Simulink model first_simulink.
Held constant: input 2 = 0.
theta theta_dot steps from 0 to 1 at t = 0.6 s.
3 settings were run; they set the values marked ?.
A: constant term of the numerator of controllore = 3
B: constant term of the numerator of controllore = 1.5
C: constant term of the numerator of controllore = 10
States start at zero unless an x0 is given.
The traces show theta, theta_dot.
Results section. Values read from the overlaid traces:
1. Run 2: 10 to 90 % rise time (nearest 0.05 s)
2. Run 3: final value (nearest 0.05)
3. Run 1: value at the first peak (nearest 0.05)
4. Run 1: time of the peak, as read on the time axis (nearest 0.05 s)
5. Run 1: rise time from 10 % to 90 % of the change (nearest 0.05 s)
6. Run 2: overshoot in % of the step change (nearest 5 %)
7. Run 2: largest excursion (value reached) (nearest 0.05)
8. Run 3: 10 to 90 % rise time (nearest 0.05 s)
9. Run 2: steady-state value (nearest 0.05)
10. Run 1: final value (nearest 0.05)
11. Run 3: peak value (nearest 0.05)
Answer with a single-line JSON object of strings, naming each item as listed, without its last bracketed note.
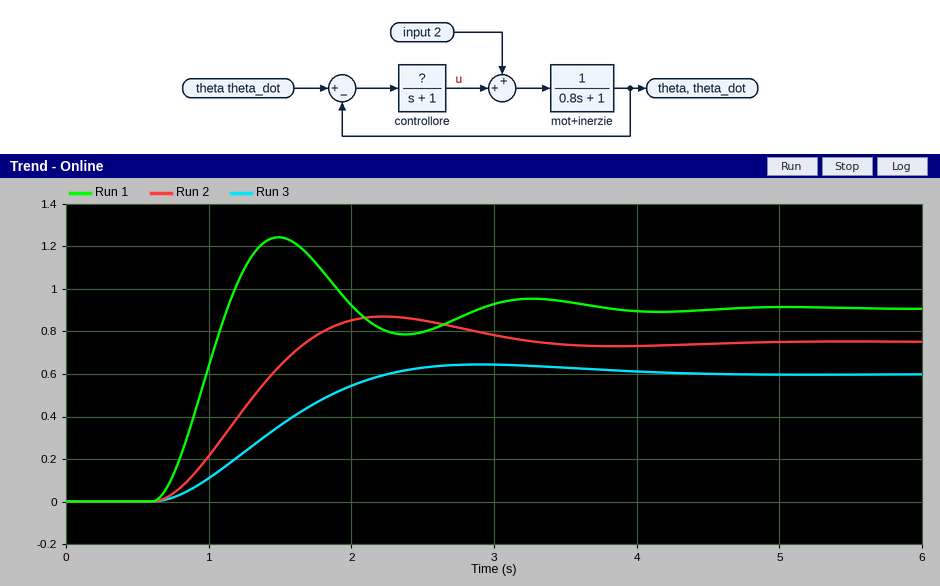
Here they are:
{"Run 2: 10 to 90 % rise time": "0.75 s", "Run 3: final value": "0.60", "Run 1: value at the first peak": "1.25", "Run 1: time of the peak, as read on the time axis": "1.50 s", "Run 1: rise time from 10 % to 90 % of the change": "0.35 s", "Run 2: overshoot in % of the step change": "15 %", "Run 2: largest excursion (value reached)": "0.85", "Run 3: 10 to 90 % rise time": "1.10 s", "Run 2: steady-state value": "0.75", "Run 1: final value": "0.90", "Run 3: peak value": "0.65"}
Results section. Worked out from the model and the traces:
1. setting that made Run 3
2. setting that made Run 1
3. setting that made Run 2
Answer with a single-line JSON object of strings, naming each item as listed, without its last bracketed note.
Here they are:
{"setting that made Run 3": "B", "setting that made Run 1": "C", "setting that made Run 2": "A"}
